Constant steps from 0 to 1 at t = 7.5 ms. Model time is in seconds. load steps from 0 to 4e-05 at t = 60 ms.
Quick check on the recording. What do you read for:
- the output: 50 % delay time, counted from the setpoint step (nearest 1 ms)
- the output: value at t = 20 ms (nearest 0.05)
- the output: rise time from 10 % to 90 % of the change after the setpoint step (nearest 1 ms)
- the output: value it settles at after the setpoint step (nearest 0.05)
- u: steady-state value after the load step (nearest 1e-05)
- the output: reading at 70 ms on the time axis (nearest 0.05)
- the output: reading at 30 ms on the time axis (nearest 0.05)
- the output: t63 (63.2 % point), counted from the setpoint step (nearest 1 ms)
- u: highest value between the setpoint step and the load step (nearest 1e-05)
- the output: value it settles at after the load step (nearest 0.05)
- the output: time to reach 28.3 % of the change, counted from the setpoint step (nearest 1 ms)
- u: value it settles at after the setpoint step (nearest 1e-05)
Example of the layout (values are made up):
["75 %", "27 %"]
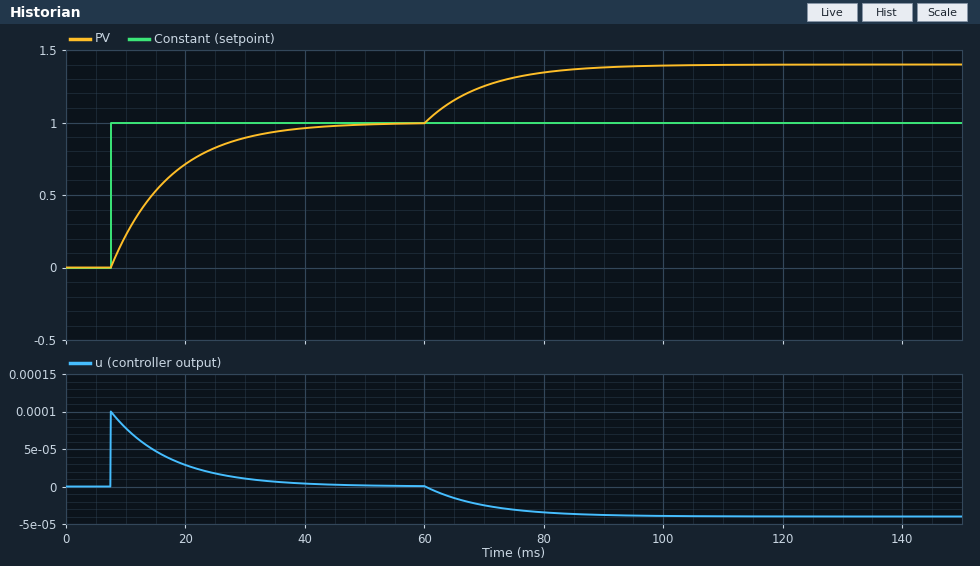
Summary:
["7 ms", "0.70", "22 ms", "1.00", "-0.00004", "1.25", "0.90", "10 ms", "0.00010", "1.40", "3 ms", "0.00000"]
